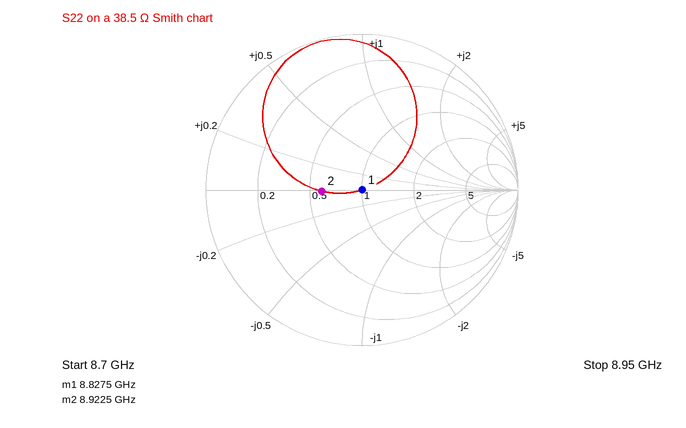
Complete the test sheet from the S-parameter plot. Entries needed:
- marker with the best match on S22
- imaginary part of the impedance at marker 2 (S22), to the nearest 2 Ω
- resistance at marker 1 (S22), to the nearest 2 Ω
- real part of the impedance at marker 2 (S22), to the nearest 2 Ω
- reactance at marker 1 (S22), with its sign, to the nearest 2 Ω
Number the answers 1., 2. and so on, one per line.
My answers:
1. marker 1
2. 0 Ω
3. 38 Ω
4. 22 Ω
5. 0 Ω
